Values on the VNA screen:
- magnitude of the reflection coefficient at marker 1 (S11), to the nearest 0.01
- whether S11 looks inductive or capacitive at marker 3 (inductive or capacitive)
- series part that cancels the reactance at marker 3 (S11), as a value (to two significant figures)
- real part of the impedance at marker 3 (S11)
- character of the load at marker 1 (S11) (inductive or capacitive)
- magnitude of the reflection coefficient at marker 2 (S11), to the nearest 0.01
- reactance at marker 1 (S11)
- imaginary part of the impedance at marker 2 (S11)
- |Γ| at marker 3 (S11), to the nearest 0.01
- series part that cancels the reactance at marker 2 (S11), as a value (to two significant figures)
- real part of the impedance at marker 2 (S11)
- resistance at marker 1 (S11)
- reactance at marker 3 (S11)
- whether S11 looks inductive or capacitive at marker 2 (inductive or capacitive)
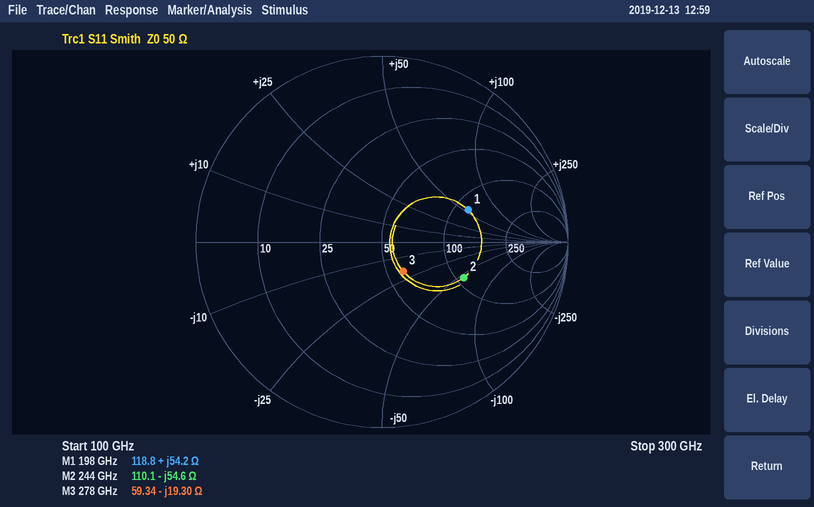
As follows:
0.49
capacitive
11 pH
59.34 Ω
inductive
0.48
+54.2 Ω
-54.6 Ω
0.19
36 pH
110.1 Ω
118.8 Ω
-19.30 Ω
capacitive
